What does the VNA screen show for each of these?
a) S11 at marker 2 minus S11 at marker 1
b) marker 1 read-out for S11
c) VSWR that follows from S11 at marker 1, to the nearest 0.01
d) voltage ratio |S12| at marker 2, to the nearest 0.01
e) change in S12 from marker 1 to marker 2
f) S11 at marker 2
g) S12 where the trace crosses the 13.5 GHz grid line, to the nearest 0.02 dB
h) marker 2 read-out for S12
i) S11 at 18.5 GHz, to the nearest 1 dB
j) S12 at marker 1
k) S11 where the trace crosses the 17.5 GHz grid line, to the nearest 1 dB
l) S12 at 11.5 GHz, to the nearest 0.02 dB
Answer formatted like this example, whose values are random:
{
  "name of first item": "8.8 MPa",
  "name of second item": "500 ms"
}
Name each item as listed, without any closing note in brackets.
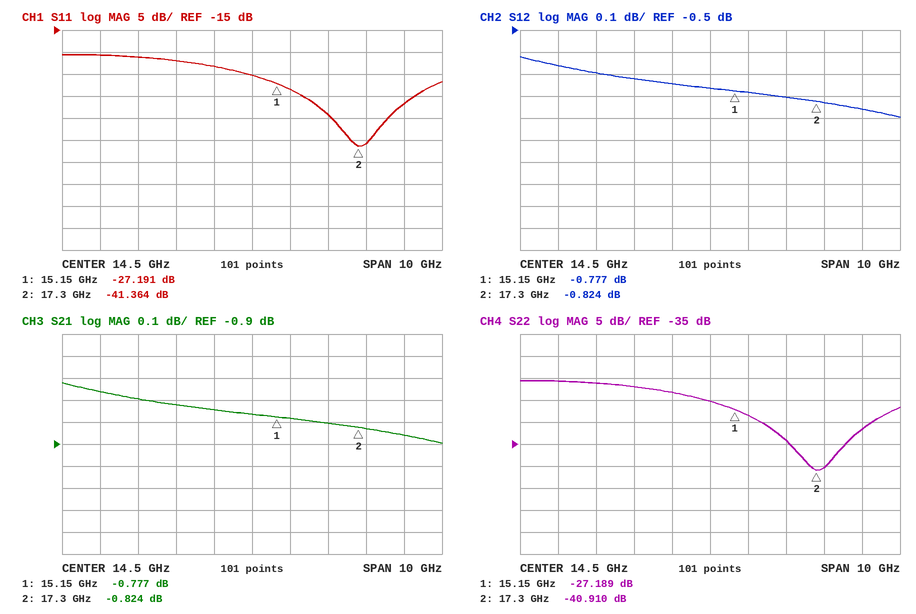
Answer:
{
  "S11 at marker 2 minus S11 at marker 1": "-14.173 dB",
  "marker 1 read-out for S11": "-27.191 dB",
  "VSWR that follows from S11 at marker 1, to the nearest 0.01": "1.09",
  "voltage ratio |S12| at marker 2, to the nearest 0.01": "0.91",
  "change in S12 from marker 1 to marker 2": "-0.047 dB",
  "S11 at marker 2": "-41.364 dB",
  "S12 where the trace crosses the 13.5 GHz grid line, to the nearest 0.02 dB": "-0.74 dB",
  "marker 2 read-out for S12": "-0.824 dB",
  "S11 at 18.5 GHz, to the nearest 1 dB": "-32 dB",
  "S12 at marker 1": "-0.777 dB",
  "S11 where the trace crosses the 17.5 GHz grid line, to the nearest 1 dB": "-41 dB",
  "S12 at 11.5 GHz, to the nearest 0.02 dB": "-0.70 dB"
}
